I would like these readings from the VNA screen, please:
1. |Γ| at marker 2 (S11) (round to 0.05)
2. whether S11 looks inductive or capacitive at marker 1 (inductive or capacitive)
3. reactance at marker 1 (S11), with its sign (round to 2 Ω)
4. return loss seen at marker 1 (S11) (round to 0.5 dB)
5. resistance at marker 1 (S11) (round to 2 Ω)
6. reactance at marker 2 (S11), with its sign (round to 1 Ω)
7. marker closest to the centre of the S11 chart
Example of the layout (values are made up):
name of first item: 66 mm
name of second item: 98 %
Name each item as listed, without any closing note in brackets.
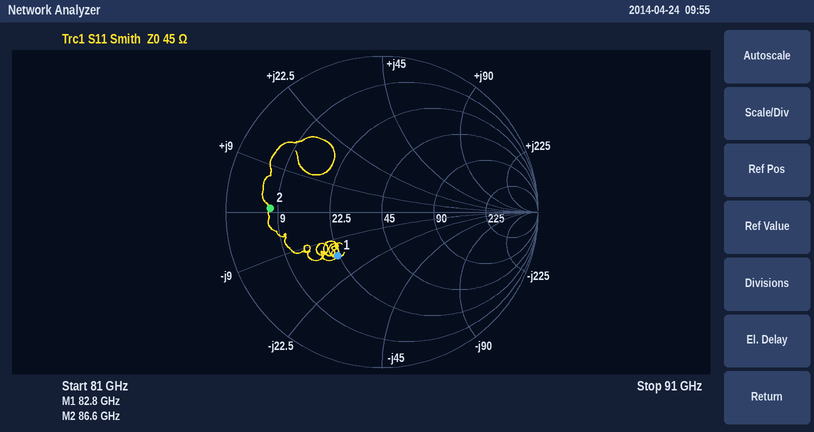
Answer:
|Γ| at marker 2 (S11): 0.70
whether S11 looks inductive or capacitive at marker 1: capacitive
reactance at marker 1 (S11), with its sign: -14 Ω
return loss seen at marker 1 (S11): 8.0 dB
resistance at marker 1 (S11): 22 Ω
reactance at marker 2 (S11), with its sign: +1 Ω
marker closest to the centre of the S11 chart: marker 1
